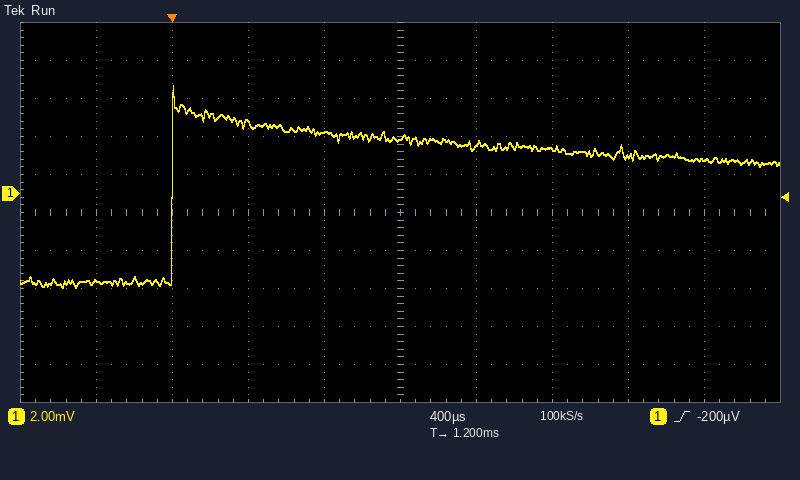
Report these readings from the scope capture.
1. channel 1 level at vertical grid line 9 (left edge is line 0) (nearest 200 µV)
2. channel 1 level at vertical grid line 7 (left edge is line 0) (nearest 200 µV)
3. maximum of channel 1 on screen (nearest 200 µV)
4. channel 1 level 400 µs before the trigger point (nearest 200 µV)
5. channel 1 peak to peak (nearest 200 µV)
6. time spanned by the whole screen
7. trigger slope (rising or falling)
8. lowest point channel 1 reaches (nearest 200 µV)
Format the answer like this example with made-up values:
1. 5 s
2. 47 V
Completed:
1. 1.8 mV
2. 2.4 mV
3. 5.6 mV
4. -4.6 mV
5. 10.6 mV
6. 4 ms
7. rising
8. -5.0 mV
